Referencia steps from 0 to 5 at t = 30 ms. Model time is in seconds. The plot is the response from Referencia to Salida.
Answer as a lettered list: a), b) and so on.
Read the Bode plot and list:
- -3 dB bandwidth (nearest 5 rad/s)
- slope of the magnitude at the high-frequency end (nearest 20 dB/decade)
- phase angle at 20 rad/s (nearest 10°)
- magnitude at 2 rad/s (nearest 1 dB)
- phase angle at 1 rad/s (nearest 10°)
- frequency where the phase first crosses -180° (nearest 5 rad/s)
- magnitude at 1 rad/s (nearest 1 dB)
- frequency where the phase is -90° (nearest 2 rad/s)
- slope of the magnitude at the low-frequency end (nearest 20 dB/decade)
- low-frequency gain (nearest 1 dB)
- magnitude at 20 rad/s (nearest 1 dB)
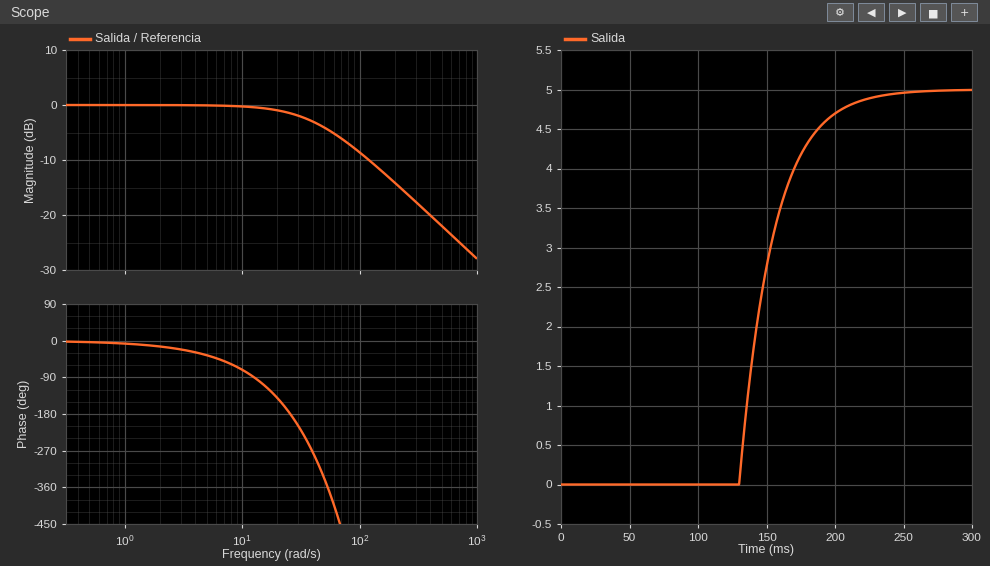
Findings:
a) 40 rad/s
b) -20 dB/decade
c) -140°
d) 0 dB
e) -10°
f) 25 rad/s
g) 0 dB
h) 12 rad/s
i) 0 dB/decade
j) 0 dB
k) -1 dB
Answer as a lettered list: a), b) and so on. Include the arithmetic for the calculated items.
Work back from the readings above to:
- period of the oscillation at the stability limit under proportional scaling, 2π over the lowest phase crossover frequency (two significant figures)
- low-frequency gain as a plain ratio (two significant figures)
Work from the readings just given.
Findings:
a) 2π / 25 = 0.25 s
b) 10^(0 / 20) = 1.0
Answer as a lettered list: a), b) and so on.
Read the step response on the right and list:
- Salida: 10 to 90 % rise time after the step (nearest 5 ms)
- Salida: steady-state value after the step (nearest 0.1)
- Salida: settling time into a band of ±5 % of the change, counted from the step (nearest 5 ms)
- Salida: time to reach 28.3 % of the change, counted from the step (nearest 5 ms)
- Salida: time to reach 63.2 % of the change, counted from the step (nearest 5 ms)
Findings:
a) 55 ms
b) 5.0
c) 175 ms
d) 110 ms
e) 125 ms
